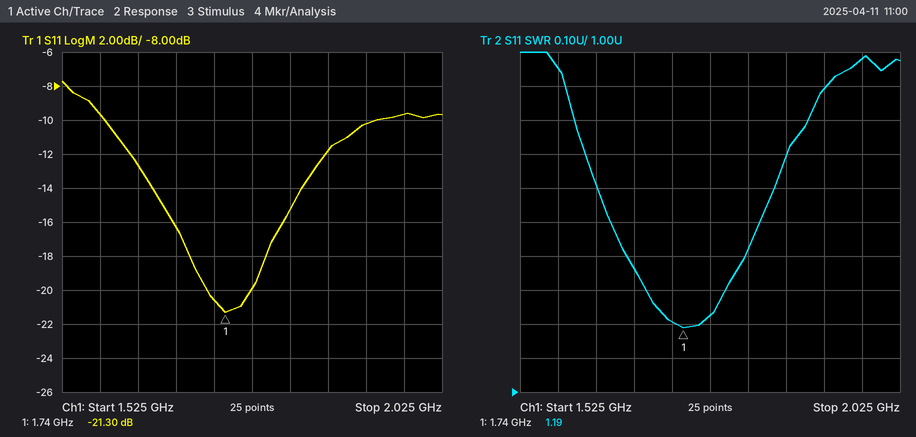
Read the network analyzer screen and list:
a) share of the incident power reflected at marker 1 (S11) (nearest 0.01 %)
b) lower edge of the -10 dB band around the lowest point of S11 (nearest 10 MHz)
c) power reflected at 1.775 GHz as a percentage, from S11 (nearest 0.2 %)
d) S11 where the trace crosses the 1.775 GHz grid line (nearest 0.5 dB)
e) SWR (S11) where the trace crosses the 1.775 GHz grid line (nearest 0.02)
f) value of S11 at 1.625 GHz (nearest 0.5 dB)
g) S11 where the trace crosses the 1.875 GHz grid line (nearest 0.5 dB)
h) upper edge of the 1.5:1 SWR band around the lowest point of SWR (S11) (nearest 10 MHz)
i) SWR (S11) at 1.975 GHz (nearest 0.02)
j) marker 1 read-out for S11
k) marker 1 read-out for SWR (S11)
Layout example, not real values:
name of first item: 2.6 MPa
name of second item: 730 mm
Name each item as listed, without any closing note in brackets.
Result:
share of the incident power reflected at marker 1 (S11): 0.74 %
lower edge of the -10 dB band around the lowest point of S11: 1.58 GHz
power reflected at 1.775 GHz as a percentage, from S11: 1.0 %
S11 where the trace crosses the 1.775 GHz grid line: -20.0 dB
SWR (S11) where the trace crosses the 1.775 GHz grid line: 1.22
value of S11 at 1.625 GHz: -12.5 dB
S11 where the trace crosses the 1.875 GHz grid line: -12.0 dB
upper edge of the 1.5:1 SWR band around the lowest point of SWR (S11): 1.84 GHz
SWR (S11) at 1.975 GHz: 1.98
marker 1 read-out for S11: -21.30 dB
marker 1 read-out for SWR: 1.19
